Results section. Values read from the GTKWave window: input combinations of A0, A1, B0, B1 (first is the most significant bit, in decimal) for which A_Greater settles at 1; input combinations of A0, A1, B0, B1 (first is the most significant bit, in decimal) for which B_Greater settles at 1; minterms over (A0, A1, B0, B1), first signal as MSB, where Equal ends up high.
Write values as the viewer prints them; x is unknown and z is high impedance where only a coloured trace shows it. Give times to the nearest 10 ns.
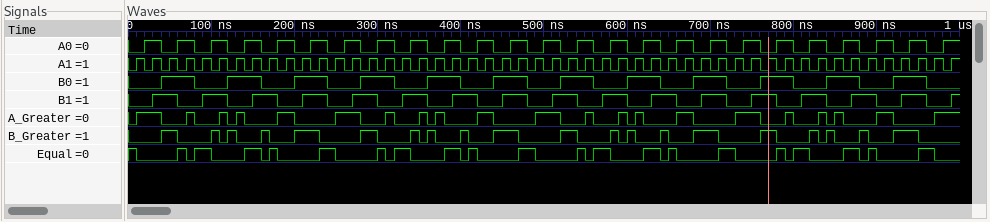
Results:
4, 6, 8, 12, 13, 14
1, 2, 3, 7, 9, 11
0, 5, 10, 15
